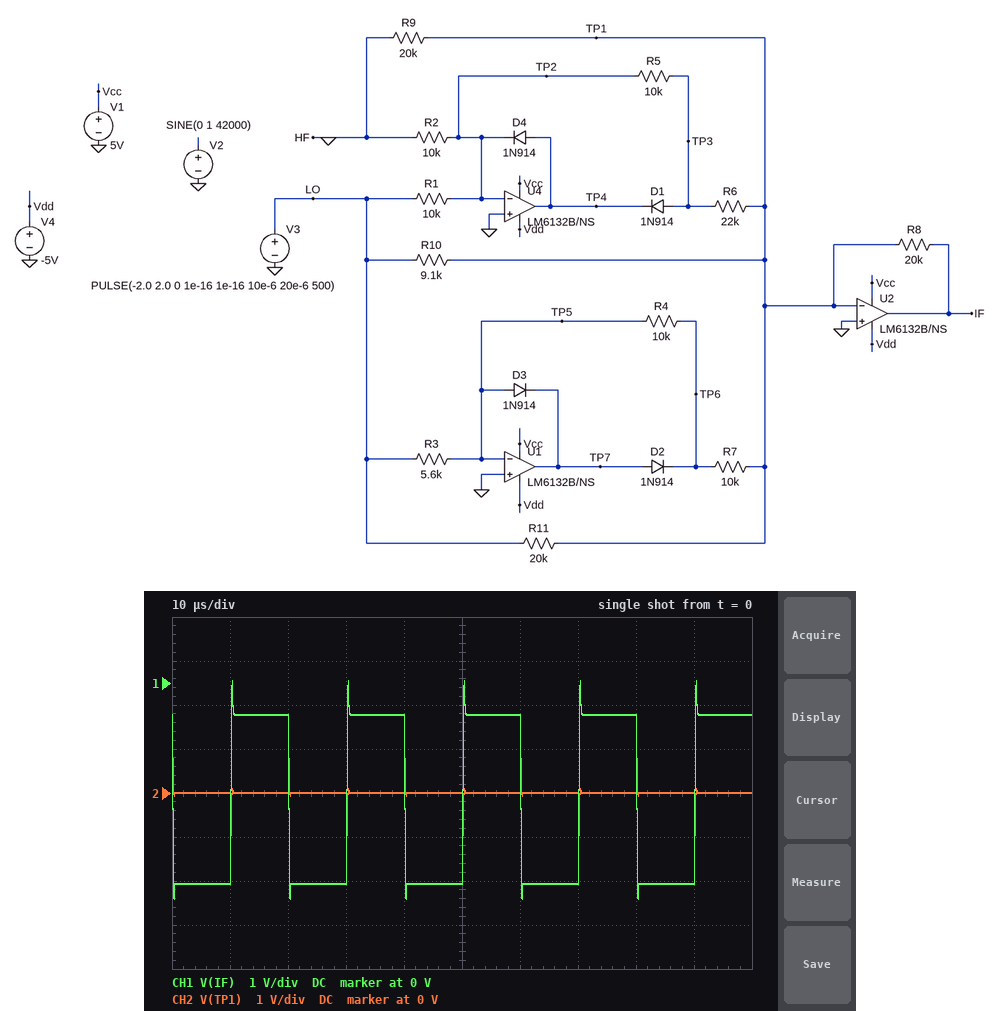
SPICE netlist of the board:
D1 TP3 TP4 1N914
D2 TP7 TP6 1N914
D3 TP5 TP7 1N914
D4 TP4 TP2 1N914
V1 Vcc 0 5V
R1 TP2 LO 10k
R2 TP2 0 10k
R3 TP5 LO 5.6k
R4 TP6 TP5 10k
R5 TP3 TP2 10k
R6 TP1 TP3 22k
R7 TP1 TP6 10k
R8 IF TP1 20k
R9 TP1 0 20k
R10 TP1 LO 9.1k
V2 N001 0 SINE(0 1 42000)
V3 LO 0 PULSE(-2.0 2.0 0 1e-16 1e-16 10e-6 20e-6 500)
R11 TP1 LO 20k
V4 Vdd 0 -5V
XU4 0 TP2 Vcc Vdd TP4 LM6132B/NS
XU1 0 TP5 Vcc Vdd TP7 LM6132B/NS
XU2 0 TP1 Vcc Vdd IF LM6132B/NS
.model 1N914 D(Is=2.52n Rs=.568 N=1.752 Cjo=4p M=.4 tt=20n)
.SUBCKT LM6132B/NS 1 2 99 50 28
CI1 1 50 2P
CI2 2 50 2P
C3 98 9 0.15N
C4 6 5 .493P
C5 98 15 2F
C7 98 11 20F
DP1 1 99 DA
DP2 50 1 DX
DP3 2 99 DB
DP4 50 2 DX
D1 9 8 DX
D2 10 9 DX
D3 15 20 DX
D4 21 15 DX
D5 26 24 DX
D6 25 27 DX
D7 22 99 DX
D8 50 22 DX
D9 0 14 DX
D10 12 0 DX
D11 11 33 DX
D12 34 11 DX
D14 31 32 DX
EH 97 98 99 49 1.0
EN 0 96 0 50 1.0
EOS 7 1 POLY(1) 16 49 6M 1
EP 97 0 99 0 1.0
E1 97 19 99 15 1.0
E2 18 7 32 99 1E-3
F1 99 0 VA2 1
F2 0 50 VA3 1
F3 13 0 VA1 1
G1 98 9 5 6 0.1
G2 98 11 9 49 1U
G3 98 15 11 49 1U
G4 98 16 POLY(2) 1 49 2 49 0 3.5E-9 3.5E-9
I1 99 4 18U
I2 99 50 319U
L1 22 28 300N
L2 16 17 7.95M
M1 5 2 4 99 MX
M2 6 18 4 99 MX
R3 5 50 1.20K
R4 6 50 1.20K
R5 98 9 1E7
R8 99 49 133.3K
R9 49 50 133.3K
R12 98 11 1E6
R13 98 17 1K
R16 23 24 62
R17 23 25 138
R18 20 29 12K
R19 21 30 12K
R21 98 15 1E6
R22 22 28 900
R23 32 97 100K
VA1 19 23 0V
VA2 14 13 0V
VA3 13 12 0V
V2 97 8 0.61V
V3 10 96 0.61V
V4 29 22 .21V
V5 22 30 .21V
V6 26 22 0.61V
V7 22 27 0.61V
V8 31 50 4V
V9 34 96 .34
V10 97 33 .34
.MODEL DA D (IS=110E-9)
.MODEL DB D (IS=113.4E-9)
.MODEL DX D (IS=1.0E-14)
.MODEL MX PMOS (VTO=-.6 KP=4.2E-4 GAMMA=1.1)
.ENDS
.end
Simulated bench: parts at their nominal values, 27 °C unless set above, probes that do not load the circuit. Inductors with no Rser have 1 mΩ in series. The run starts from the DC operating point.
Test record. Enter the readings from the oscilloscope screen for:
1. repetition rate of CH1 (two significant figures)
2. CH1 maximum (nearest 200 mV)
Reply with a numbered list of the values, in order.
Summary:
1. 50 kHz
2. 0 V
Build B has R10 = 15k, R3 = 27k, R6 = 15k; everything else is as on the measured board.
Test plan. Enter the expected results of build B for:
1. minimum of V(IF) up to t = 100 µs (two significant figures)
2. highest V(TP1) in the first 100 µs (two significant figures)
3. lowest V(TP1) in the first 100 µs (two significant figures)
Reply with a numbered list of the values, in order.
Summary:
1. -2.0 V
2. 1.3 V
3. -1.3 V
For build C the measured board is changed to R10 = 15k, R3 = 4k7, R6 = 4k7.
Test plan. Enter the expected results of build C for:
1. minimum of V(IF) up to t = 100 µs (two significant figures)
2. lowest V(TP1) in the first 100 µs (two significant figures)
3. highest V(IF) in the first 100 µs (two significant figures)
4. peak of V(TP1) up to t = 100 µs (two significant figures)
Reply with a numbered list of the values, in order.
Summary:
1. -5.0 V
2. -920 mV
3. 5.0 V
4. 1.1 V
